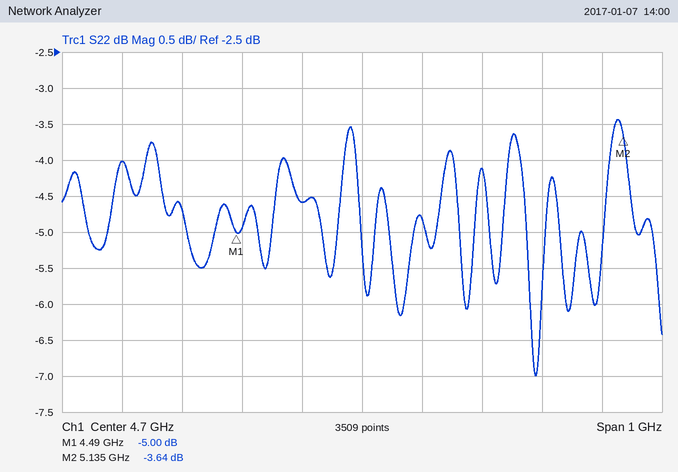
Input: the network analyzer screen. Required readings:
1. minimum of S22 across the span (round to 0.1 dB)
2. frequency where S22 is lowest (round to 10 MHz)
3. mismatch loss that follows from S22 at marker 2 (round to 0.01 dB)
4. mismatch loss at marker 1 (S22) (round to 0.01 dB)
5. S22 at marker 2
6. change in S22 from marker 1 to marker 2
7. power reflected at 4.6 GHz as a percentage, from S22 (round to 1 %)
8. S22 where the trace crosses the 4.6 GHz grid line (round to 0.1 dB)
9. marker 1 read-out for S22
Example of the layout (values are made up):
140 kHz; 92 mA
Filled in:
-7.0 dB; 4.99 GHz; 2.46 dB; 1.65 dB; -3.64 dB; 1.36 dB; 35 %; -4.6 dB; -5.00 dB
